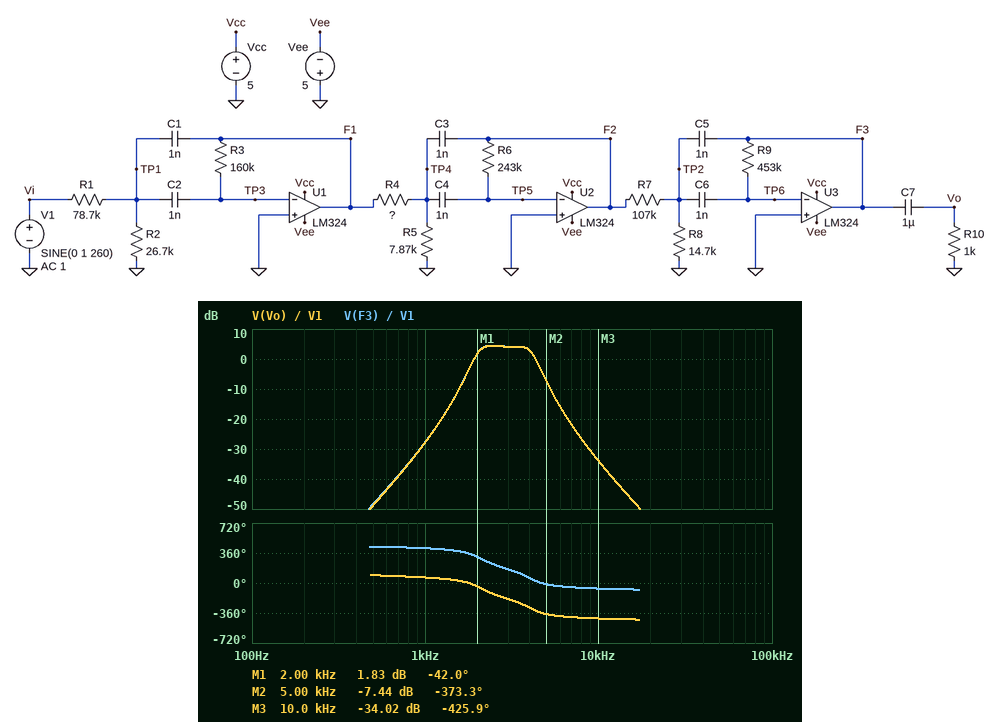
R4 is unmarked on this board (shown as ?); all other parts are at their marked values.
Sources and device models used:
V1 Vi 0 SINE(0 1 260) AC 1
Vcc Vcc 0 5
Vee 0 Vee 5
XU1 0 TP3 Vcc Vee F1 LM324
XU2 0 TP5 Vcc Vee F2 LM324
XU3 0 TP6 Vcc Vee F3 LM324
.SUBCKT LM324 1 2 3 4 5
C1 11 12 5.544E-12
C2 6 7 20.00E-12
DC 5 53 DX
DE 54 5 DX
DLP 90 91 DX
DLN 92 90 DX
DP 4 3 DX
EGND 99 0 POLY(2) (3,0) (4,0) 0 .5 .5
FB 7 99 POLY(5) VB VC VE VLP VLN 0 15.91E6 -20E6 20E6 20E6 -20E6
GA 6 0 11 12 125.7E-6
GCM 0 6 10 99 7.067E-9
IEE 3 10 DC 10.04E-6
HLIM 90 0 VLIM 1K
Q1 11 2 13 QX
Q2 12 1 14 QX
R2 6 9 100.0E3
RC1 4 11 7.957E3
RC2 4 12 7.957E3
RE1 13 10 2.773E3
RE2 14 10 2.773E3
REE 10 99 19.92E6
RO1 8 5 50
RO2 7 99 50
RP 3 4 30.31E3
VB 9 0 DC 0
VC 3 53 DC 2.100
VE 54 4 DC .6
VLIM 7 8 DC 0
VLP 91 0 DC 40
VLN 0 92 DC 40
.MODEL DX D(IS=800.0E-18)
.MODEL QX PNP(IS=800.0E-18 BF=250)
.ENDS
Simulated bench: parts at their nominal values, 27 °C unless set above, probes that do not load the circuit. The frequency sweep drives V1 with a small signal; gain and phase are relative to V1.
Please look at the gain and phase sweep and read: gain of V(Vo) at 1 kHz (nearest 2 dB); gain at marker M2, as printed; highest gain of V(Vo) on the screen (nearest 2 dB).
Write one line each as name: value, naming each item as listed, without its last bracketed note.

gain of V(Vo) at 1 kHz: -28 dB
gain at marker M2, as printed: -7.44 dB
highest gain of V(Vo) on the screen: 4 dB
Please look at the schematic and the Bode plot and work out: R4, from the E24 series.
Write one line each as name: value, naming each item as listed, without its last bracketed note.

R4, from the E24 series: 30 kΩ
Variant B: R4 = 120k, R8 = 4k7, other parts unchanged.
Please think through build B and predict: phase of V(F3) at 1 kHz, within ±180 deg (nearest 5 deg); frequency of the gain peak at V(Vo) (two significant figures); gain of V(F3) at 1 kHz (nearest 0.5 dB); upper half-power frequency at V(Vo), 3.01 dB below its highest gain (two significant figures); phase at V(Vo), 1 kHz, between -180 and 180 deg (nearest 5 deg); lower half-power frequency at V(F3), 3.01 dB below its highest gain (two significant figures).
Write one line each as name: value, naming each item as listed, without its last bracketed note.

phase of V(F3) at 1 kHz, within ±180 deg: 65 deg
frequency of the gain peak at V(Vo): 3.5 kHz
gain of V(F3) at 1 kHz: -48.5 dB
upper half-power frequency at V(Vo), 3.01 dB below its highest gain: 3.8 kHz
phase at V(Vo), 1 kHz, between -180 and 180 deg: 75 deg
lower half-power frequency at V(F3), 3.01 dB below its highest gain: 3.2 kHz
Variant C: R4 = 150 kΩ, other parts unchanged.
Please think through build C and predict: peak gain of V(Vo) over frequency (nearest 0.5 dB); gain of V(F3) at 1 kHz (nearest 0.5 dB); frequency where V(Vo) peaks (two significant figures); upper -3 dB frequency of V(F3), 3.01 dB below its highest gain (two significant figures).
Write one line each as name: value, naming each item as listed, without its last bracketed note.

peak gain of V(Vo) over frequency: -7.0 dB
gain of V(F3) at 1 kHz: -40.0 dB
frequency where V(Vo) peaks: 3.0 kHz
upper -3 dB frequency of V(F3), 3.01 dB below its highest gain: 3.8 kHz
